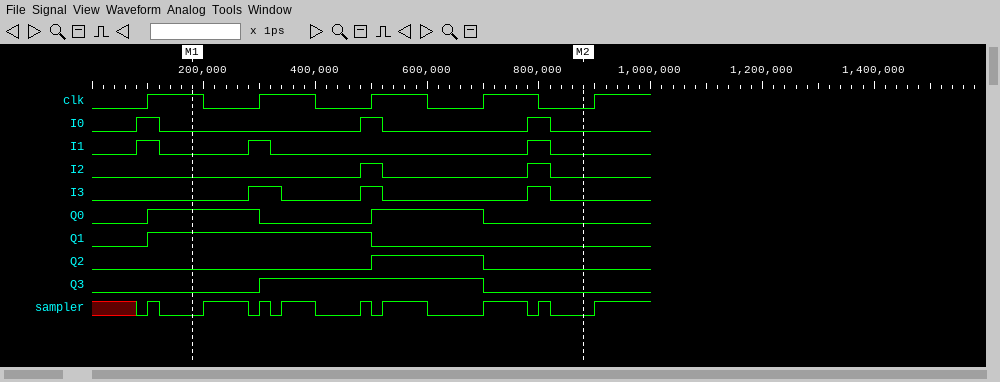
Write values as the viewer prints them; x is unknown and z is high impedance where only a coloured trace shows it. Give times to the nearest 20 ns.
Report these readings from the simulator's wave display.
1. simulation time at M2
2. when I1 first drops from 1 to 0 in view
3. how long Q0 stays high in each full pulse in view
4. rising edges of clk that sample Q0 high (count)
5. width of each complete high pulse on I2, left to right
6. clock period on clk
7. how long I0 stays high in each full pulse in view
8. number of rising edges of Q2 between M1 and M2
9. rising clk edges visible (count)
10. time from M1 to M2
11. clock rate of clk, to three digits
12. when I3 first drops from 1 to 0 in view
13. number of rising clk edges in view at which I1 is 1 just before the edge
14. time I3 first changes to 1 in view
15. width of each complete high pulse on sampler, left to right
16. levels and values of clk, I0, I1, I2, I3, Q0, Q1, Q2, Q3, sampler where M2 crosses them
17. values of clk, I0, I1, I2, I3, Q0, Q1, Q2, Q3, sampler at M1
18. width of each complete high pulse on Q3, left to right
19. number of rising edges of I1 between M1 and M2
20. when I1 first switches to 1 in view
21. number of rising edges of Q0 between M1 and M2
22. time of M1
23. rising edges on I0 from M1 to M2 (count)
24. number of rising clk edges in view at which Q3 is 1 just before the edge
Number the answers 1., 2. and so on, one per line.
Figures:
1. 880 ns
2. 120 ns
3. 200 ns, 200 ns
4. 2
5. 40 ns, 40 ns
6. 200 ns
7. 40 ns, 40 ns, 40 ns
8. 1
9. 5
10. 700 ns
11. 5.00 MHz
12. 340 ns
13. 2
14. 280 ns
15. 20 ns, 80 ns, 20 ns, 60 ns, 20 ns, 80 ns, 80 ns, 20 ns
16. clk=0, I0=0, I1=0, I2=0, I3=0, Q0=0, Q1=0, Q2=0, Q3=0, sampler=0
17. clk=1, I0=0, I1=0, I2=0, I3=0, Q0=1, Q1=1, Q2=0, Q3=0, sampler=0
18. 400 ns
19. 2
20. 80 ns
21. 1
22. 180 ns
23. 2
24. 2
